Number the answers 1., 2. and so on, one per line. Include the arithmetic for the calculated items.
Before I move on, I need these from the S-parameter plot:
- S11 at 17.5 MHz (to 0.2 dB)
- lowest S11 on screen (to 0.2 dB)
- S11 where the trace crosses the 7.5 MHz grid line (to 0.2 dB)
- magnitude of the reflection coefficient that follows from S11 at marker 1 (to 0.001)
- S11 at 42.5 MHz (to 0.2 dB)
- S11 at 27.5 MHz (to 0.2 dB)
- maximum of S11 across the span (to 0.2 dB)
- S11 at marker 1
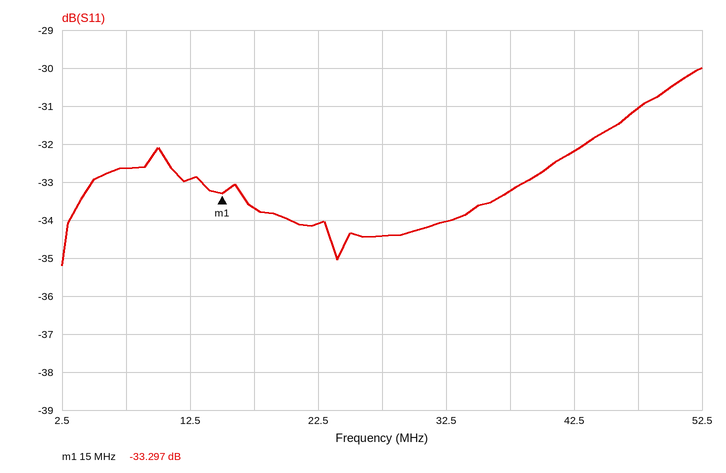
1. -33.6 dB
2. -35.2 dB
3. -32.6 dB
4. 10^(-33.297/20) ≈ 0.022
5. -32.2 dB
6. -34.4 dB
7. -30.0 dB
8. -33.297 dB
